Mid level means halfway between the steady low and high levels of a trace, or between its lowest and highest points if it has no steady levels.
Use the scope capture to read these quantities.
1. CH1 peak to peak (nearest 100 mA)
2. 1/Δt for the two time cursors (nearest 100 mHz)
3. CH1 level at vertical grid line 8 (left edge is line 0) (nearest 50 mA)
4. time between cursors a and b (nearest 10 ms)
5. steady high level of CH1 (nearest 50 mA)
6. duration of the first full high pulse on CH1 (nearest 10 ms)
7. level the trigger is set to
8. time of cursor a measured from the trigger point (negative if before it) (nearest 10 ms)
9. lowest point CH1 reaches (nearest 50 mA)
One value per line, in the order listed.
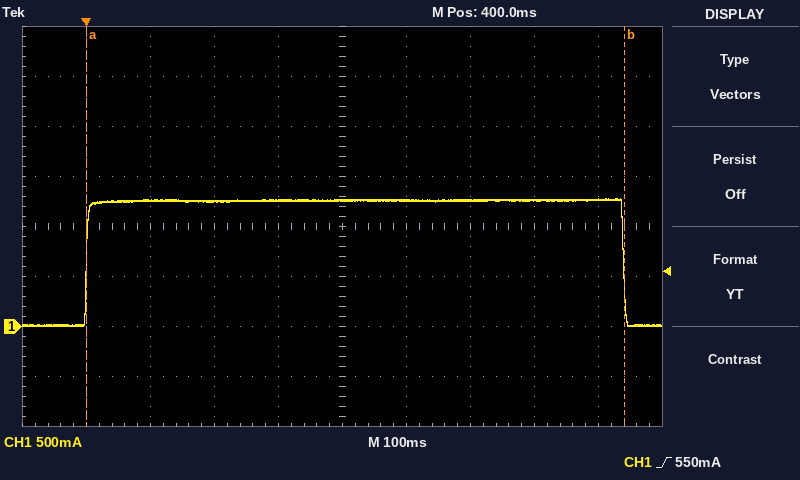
1.30 A
1.2 Hz
1.25 A
840 ms
1.25 A
840 ms
550 mA
0 ms
0 mA
